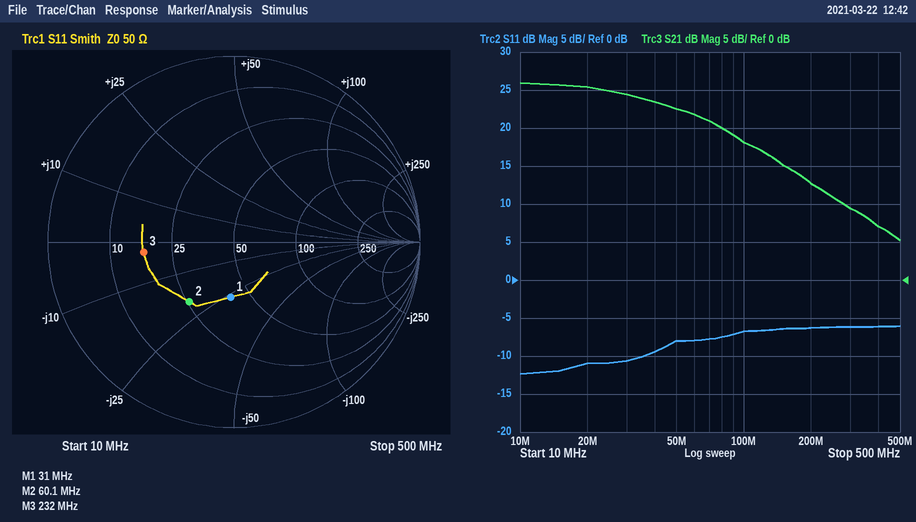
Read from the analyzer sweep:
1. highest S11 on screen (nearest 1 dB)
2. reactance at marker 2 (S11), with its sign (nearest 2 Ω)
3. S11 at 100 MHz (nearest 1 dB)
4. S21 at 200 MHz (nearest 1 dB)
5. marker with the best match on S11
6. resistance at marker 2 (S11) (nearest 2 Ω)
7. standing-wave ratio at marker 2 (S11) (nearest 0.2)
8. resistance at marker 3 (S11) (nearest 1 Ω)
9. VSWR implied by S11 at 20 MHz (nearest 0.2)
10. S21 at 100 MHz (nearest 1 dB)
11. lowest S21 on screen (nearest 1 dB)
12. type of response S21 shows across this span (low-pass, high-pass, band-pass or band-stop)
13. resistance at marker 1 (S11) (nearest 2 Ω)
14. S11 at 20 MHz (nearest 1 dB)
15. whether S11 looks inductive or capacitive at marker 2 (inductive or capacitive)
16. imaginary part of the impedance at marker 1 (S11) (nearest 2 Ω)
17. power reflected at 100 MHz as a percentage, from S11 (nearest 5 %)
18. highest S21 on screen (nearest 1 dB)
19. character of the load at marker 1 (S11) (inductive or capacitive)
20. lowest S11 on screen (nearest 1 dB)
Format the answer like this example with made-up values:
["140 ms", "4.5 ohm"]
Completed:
["-6 dB", "-20 Ω", "-7 dB", "13 dB", "marker 1", "26 Ω", "2.4", "17 Ω", "1.8", "18 dB", "5 dB", "low-pass", "40 Ω", "-11 dB", "capacitive", "-26 Ω", "20 %", "26 dB", "capacitive", "-12 dB"]
